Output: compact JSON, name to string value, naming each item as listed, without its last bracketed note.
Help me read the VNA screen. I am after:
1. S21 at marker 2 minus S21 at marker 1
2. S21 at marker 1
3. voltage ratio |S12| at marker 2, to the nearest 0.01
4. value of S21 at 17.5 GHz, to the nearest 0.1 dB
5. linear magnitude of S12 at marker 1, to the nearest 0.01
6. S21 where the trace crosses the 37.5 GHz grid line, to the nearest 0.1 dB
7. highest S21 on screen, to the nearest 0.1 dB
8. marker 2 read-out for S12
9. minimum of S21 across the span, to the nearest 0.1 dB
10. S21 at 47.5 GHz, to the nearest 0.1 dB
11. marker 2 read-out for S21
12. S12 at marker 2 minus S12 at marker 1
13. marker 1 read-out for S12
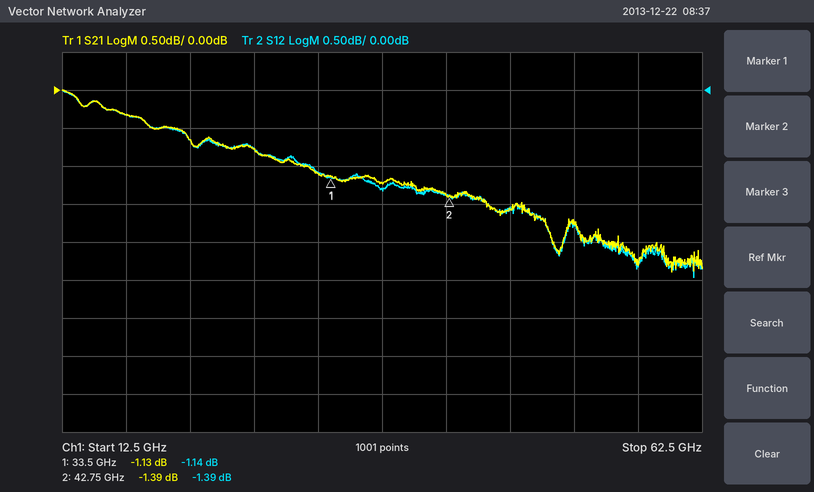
{"S21 at marker 2 minus S21 at marker 1": "-0.26 dB", "S21 at marker 1": "-1.13 dB", "voltage ratio |S12| at marker 2, to the nearest 0.01": "0.85", "value of S21 at 17.5 GHz, to the nearest 0.1 dB": "-0.3 dB", "linear magnitude of S12 at marker 1, to the nearest 0.01": "0.88", "S21 where the trace crosses the 37.5 GHz grid line, to the nearest 0.1 dB": "-1.2 dB", "highest S21 on screen, to the nearest 0.1 dB": "0.0 dB", "marker 2 read-out for S12": "-1.39 dB", "minimum of S21 across the span, to the nearest 0.1 dB": "-2.4 dB", "S21 at 47.5 GHz, to the nearest 0.1 dB": "-1.6 dB", "marker 2 read-out for S21": "-1.39 dB", "S12 at marker 2 minus S12 at marker 1": "-0.25 dB", "marker 1 read-out for S12": "-1.14 dB"}
